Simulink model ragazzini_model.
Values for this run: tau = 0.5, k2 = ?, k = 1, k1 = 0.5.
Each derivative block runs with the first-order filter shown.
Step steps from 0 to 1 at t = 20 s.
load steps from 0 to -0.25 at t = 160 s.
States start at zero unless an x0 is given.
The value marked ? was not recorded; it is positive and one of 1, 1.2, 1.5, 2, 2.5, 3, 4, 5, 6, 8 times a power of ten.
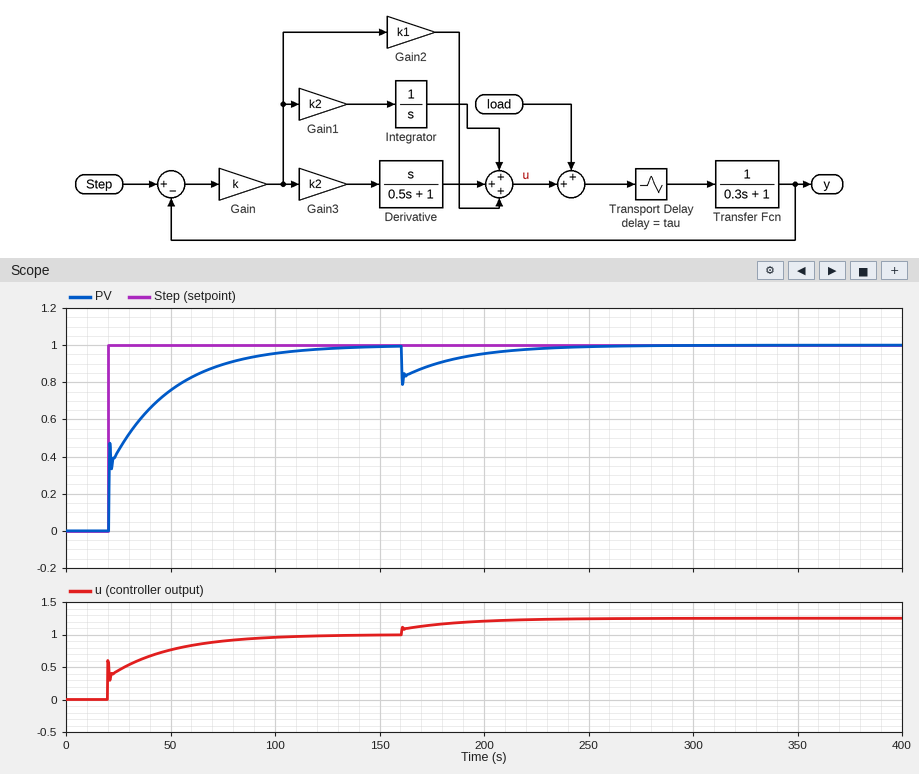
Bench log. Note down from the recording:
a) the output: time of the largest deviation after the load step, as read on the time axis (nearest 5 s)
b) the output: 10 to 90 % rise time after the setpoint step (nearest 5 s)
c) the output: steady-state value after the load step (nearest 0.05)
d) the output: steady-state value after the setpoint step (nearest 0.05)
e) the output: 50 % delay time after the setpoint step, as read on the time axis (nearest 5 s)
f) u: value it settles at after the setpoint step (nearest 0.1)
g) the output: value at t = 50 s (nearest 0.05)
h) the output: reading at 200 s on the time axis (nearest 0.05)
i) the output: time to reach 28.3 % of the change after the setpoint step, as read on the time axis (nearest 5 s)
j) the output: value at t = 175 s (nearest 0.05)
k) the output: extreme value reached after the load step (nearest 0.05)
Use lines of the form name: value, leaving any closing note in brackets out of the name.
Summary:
the output: time of the largest deviation after the load step, as read on the time axis: 160 s
the output: 10 to 90 % rise time after the setpoint step: 55 s
the output: steady-state value after the load step: 1.00
the output: steady-state value after the setpoint step: 1.00
the output: 50 % delay time after the setpoint step, as read on the time axis: 30 s
u: value it settles at after the setpoint step: 1.0
the output: value at t = 50 s: 0.75
the output: reading at 200 s on the time axis: 0.95
the output: time to reach 28.3 % of the change after the setpoint step, as read on the time axis: 20 s
the output: value at t = 175 s: 0.90
the output: extreme value reached after the load step: 0.80
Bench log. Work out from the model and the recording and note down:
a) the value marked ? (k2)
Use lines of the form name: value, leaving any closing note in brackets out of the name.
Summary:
the value marked ?: 0.05
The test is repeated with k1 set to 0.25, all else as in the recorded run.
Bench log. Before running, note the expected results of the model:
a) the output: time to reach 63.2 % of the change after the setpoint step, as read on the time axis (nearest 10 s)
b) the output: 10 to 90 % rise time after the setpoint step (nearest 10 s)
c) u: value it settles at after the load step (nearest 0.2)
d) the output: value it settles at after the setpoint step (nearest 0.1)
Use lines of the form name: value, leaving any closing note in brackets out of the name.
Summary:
the output: time to reach 63.2 % of the change after the setpoint step, as read on the time axis: 40 s
the output: 10 to 90 % rise time after the setpoint step: 50 s
u: value it settles at after the load step: 1.2
the output: value it settles at after the setpoint step: 1.0
